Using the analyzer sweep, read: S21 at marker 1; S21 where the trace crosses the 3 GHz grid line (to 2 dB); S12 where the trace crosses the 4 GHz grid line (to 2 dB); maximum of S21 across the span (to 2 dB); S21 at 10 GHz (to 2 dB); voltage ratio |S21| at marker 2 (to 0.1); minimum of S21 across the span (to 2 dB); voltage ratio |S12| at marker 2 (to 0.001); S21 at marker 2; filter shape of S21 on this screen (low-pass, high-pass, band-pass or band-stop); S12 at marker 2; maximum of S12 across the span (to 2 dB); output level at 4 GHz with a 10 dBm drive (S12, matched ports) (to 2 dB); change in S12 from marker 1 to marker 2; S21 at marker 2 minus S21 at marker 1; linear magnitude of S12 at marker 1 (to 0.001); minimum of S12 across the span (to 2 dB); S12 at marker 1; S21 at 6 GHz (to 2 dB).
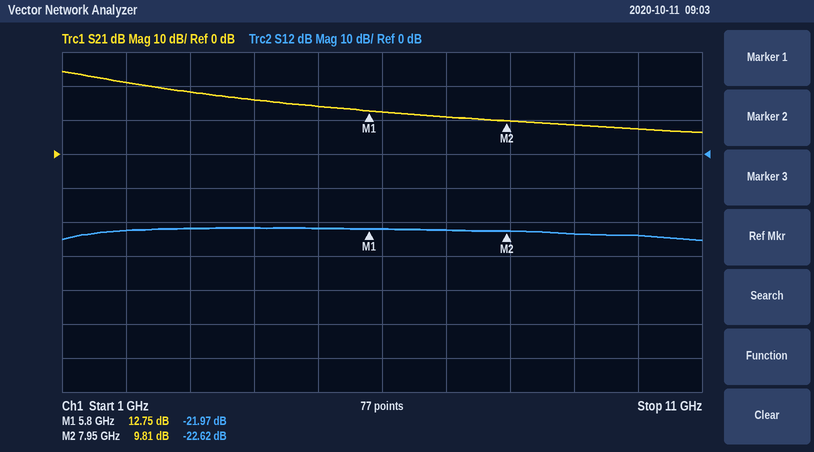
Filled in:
12.75 dB
18 dB
-22 dB
24 dB
8 dB
3.1
6 dB
0.074
9.81 dB
low-pass
-22.62 dB
-22 dB
-12 dBm
-0.65 dB
-2.94 dB
0.080
-26 dB
-21.97 dB
12 dB
